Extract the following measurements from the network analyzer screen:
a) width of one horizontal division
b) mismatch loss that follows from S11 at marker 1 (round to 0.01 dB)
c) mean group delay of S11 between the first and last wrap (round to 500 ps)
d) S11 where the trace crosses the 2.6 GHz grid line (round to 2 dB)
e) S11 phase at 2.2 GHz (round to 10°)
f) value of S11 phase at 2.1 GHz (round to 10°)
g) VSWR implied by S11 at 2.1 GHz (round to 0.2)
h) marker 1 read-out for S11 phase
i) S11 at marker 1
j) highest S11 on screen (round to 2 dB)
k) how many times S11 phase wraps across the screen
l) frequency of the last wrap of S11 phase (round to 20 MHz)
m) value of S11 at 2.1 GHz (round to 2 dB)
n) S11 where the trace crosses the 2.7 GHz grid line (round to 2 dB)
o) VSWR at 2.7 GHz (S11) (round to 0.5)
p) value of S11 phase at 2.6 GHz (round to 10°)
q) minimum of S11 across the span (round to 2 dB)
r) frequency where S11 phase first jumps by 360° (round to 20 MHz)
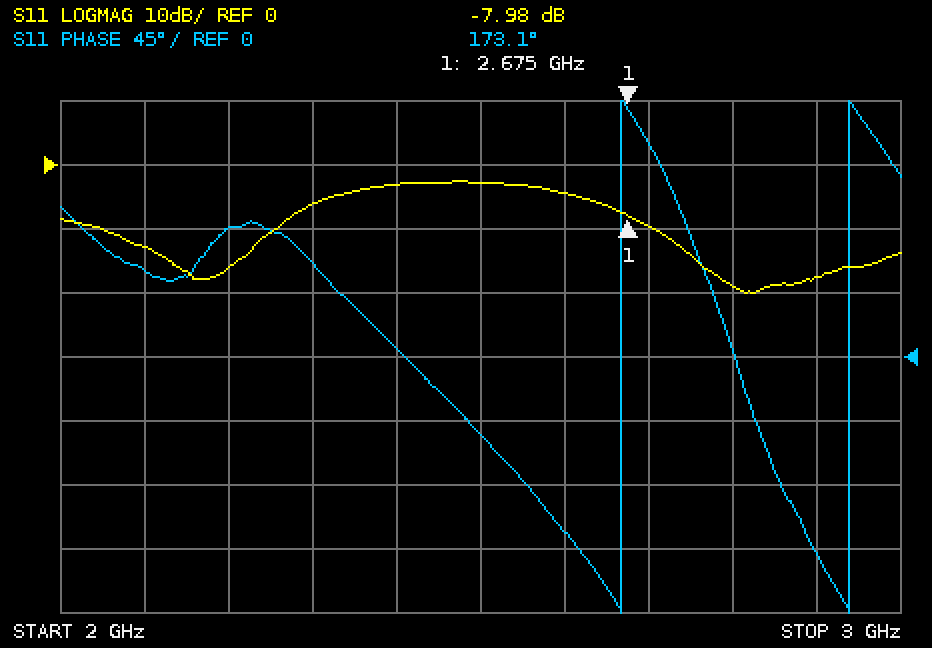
100 MHz
0.75 dB
3.5 ns
-4 dB
90°
60°
1.6
173.1°
-7.98 dB
-2 dB
2
2.94 GHz
-12 dB
-10 dB
2.0
-120°
-20 dB
2.66 GHz
